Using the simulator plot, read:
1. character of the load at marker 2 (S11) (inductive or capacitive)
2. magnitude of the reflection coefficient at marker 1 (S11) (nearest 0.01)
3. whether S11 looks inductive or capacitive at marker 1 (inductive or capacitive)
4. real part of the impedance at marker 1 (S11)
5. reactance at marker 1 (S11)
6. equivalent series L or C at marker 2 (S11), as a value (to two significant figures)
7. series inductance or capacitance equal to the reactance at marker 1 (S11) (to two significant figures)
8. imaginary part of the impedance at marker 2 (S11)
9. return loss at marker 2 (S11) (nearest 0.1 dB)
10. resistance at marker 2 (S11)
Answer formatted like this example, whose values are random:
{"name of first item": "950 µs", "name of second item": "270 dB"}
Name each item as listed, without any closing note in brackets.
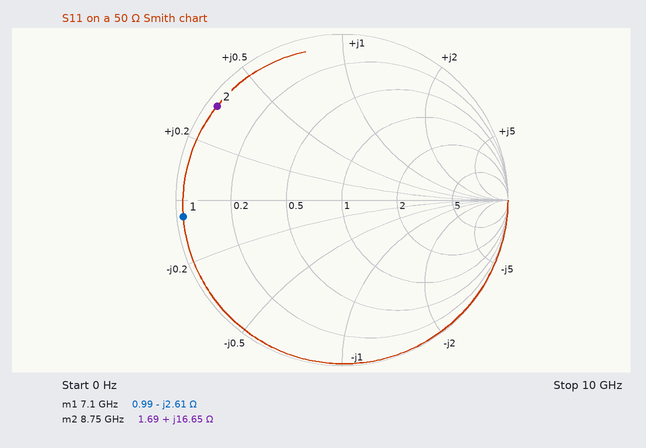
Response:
{"character of the load at marker 2 (S11)": "inductive", "magnitude of the reflection coefficient at marker 1 (S11)": "0.96", "whether S11 looks inductive or capacitive at marker 1": "capacitive", "real part of the impedance at marker 1": "0.99 Ω", "reactance at marker 1": "-2.61 Ω", "equivalent series L or C at marker 2 (S11), as a value": "300 pH", "series inductance or capacitance equal to the reactance at marker 1 (S11)": "8.6 pF", "imaginary part of the impedance at marker 2": "+16.65 Ω", "return loss at marker 2 (S11)": "0.5 dB", "resistance at marker 2": "1.69 Ω"}
